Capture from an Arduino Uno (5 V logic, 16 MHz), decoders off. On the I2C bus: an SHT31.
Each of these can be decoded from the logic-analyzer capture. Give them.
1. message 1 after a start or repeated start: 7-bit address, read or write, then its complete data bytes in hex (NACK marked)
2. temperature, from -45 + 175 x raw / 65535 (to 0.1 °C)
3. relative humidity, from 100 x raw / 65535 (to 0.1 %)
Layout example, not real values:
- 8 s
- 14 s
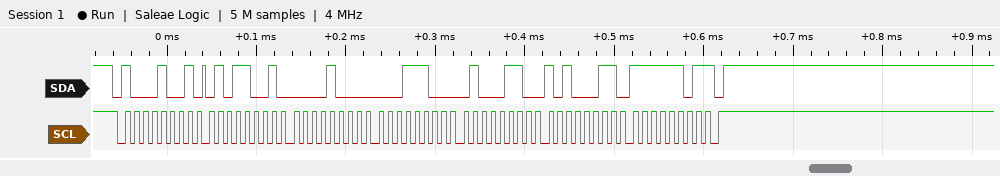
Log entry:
- 0x44 read: 59 08 1C 46 A3 FD NACK
- 15.9 °C
- 27.6 %
